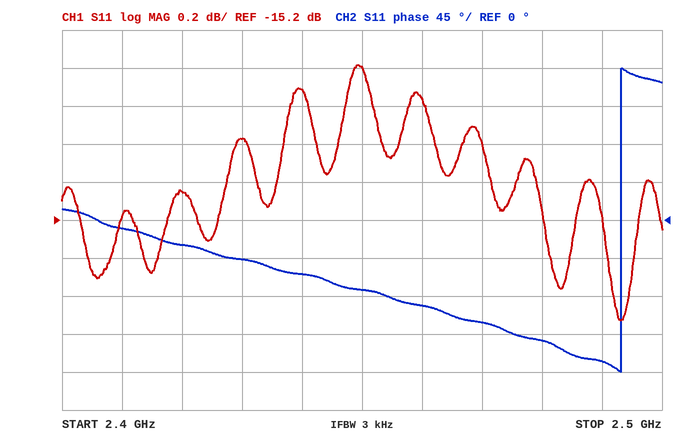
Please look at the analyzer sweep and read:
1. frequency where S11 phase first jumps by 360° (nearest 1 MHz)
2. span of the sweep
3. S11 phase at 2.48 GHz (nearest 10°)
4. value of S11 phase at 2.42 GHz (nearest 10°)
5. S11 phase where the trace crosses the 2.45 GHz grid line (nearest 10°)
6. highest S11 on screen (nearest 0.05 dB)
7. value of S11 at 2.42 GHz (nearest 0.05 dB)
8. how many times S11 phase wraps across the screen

2.493 GHz
100 MHz
-140°
-30°
-80°
-14.40 dB
-15.05 dB
1
